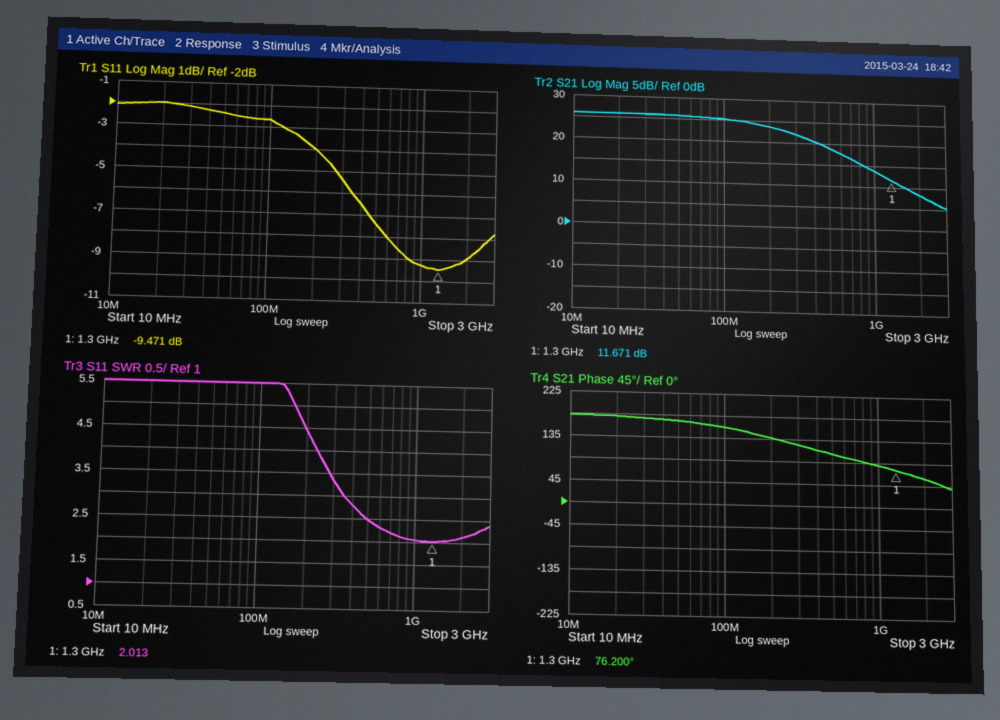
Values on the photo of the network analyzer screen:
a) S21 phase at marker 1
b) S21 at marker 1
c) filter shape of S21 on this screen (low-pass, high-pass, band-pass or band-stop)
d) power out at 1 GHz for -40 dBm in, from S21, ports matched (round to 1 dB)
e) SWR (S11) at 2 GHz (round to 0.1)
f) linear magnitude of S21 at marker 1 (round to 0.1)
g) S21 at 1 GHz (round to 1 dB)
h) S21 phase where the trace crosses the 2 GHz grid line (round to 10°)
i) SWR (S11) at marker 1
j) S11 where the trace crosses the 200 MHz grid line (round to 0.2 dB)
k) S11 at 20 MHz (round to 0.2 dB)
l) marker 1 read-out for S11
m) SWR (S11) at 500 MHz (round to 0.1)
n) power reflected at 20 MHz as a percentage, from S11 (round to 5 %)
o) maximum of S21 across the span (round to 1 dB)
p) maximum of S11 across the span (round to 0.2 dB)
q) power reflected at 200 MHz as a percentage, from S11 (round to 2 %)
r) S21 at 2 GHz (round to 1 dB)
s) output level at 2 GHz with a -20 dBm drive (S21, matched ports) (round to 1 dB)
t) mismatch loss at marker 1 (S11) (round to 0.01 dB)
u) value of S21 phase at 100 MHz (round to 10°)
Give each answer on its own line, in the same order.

76.200°
11.671 dB
low-pass
-26 dBm
2.1
3.8
14 dB
60°
2.013
-4.0 dB
-2.0 dB
-9.471 dB
2.5
65 %
26 dB
-2.0 dB
40 %
8 dB
-12 dBm
0.52 dB
160°
